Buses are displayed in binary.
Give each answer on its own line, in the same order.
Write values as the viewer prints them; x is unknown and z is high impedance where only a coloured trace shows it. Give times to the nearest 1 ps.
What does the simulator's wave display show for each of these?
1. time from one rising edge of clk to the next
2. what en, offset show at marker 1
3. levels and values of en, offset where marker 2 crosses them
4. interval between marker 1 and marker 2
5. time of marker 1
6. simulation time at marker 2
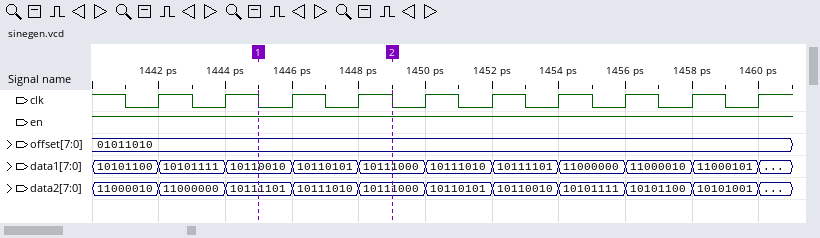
2 ps
en=1, offset=01011010
en=1, offset=01011010
4 ps
1445 ps
1449 ps
